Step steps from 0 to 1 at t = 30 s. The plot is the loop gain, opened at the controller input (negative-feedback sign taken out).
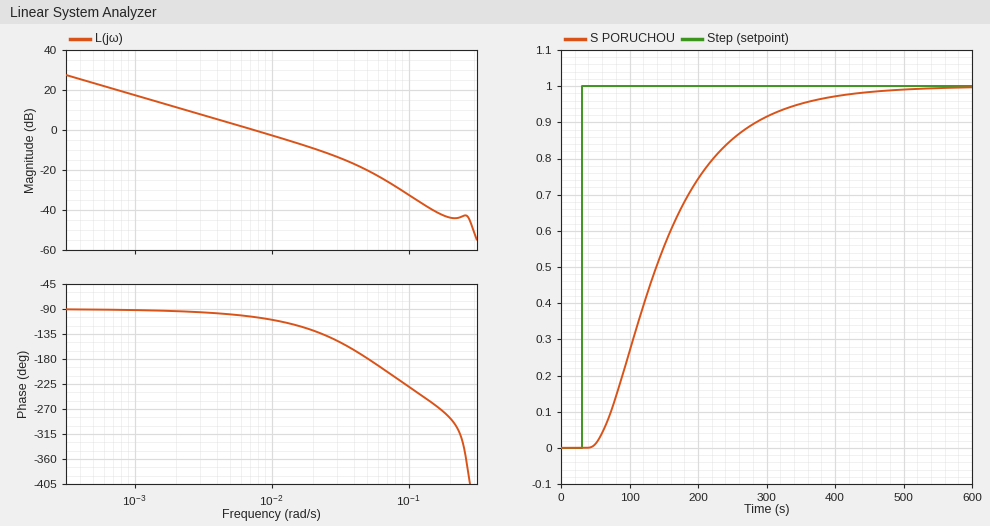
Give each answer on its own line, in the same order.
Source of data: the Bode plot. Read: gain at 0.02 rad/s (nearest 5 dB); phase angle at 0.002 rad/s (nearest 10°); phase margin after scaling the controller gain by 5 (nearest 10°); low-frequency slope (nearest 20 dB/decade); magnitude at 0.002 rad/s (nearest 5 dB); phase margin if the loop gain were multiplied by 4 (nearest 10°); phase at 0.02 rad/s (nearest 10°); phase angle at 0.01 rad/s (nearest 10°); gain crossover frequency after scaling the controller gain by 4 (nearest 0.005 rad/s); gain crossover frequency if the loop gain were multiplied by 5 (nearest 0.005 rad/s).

-10 dB
-90°
30°
-20 dB/decade
10 dB
40°
-130°
-110°
0.025 rad/s
0.030 rad/s
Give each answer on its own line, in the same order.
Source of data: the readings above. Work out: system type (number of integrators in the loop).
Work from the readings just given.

1
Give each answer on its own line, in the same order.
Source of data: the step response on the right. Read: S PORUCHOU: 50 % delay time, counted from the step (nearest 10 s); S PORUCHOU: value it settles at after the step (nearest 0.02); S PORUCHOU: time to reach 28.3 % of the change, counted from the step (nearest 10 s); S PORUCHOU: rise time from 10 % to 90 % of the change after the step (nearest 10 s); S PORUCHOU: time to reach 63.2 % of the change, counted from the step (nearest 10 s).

110 s
1.00
70 s
210 s
140 s
